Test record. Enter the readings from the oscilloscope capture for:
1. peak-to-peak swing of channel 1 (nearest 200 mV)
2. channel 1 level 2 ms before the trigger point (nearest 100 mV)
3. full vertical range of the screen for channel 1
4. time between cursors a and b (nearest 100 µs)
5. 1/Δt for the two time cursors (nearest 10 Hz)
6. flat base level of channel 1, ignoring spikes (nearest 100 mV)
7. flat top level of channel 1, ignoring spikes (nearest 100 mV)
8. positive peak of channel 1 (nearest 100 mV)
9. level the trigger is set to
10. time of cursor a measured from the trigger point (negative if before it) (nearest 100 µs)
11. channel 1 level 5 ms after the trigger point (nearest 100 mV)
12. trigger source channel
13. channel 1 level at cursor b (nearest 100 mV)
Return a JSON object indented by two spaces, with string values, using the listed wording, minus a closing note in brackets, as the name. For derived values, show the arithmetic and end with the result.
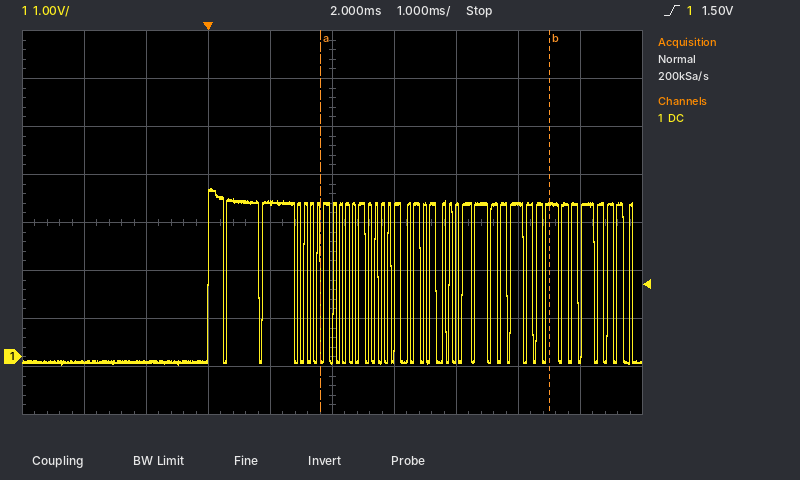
{
  "peak-to-peak swing of channel 1": "3.6 V",
  "channel 1 level 2 ms before the trigger point": "-100 mV",
  "full vertical range of the screen for channel 1": "8 V",
  "time between cursors a and b": "3.7 ms",
  "1/Δt for the two time cursors": "1 / 3.7 ms ≈ 270 Hz",
  "flat base level of channel 1, ignoring spikes": "-100 mV",
  "flat top level of channel 1, ignoring spikes": "3.2 V",
  "positive peak of channel 1": "3.5 V",
  "level the trigger is set to": "1.50 V",
  "time of cursor a measured from the trigger point (negative if before it)": "+1.8 ms",
  "channel 1 level 5 ms after the trigger point": "3.2 V",
  "trigger source channel": "channel 1",
  "channel 1 level at cursor b": "3.2 V"
}
